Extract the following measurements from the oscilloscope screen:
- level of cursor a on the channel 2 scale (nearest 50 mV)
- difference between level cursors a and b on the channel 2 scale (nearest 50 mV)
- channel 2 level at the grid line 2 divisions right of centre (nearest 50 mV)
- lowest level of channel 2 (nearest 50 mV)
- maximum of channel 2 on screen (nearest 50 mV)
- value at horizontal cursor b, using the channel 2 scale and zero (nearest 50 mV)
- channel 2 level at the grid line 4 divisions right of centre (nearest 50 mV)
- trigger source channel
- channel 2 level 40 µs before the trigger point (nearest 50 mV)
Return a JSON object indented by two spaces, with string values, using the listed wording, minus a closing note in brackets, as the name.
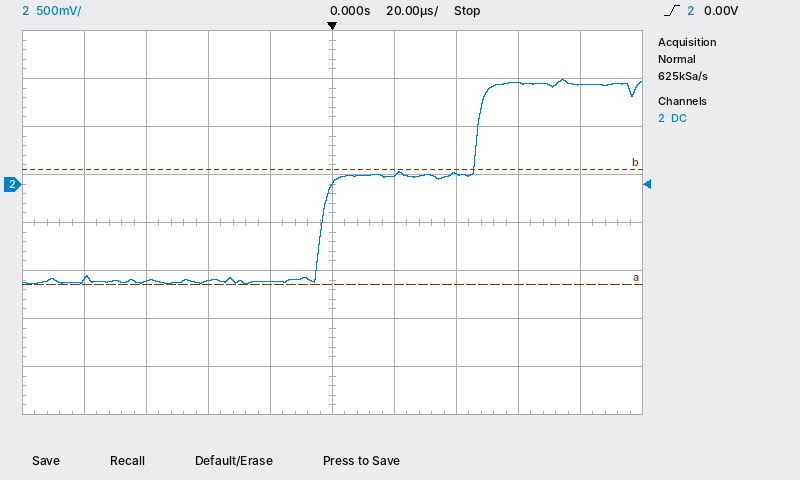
{
  "level of cursor a on the channel 2 scale": "-1.05 V",
  "difference between level cursors a and b on the channel 2 scale": "1.20 V",
  "channel 2 level at the grid line 2 divisions right of centre": "100 mV",
  "lowest level of channel 2": "-1.05 V",
  "maximum of channel 2 on screen": "1.10 V",
  "value at horizontal cursor b, using the channel 2 scale and zero": "150 mV",
  "channel 2 level at the grid line 4 divisions right of centre": "1.05 V",
  "trigger source channel": "channel 2",
  "channel 2 level 40 µs before the trigger point": "-1.00 V"
}
